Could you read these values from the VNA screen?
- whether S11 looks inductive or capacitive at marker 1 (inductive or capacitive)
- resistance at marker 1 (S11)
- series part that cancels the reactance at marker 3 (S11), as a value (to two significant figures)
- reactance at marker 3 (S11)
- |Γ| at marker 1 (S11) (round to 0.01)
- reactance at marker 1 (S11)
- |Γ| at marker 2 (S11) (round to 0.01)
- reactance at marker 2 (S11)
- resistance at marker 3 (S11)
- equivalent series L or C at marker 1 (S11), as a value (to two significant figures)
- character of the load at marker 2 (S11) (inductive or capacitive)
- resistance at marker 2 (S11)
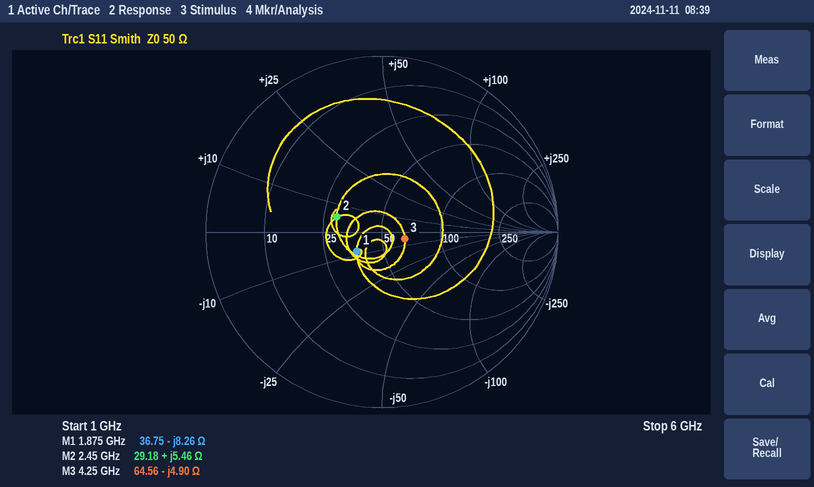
capacitive
36.75 Ω
180 pH
-4.90 Ω
0.18
-8.26 Ω
0.27
+5.46 Ω
64.56 Ω
10 pF
inductive
29.18 Ω
